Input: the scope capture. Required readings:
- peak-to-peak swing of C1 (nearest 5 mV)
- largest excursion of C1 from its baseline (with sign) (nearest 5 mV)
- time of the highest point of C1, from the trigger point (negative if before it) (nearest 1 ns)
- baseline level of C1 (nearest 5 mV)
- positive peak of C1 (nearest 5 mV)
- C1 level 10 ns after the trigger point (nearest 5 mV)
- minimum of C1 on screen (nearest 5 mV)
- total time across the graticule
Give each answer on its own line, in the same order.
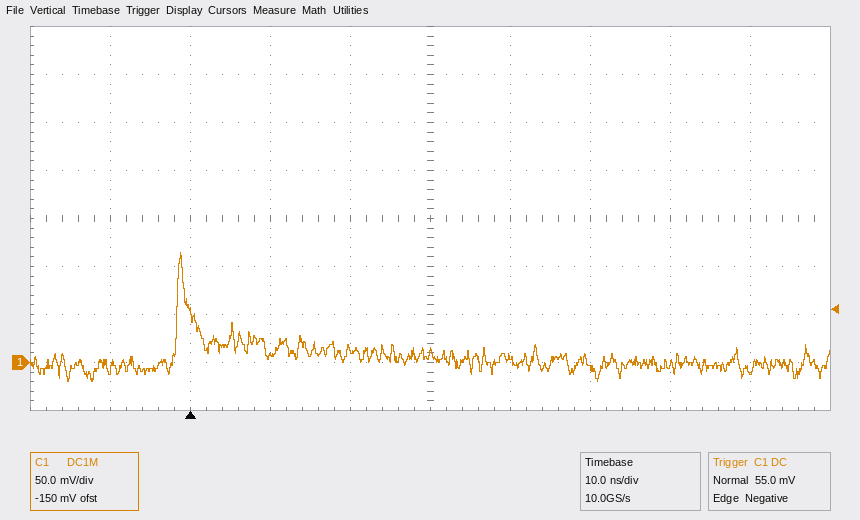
135 mV
+115 mV
-1 ns
0 mV
115 mV
5 mV
-20 mV
100 ns
